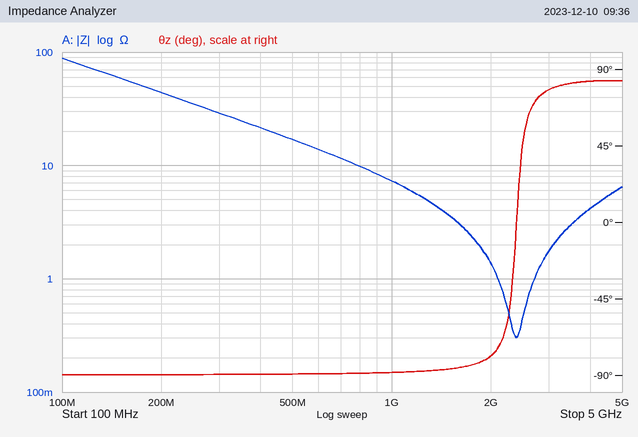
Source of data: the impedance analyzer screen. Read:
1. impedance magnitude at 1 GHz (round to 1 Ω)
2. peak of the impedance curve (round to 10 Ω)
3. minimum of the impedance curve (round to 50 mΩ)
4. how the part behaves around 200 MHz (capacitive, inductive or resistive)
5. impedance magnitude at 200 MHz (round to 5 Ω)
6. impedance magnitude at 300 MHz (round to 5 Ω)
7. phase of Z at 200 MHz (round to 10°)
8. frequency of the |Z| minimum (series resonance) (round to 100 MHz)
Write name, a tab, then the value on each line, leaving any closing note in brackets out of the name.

impedance magnitude at 1 GHz	7 Ω
peak of the impedance curve	90 Ω
minimum of the impedance curve	300 mΩ
how the part behaves around 200 MHz	capacitive
impedance magnitude at 200 MHz	45 Ω
impedance magnitude at 300 MHz	30 Ω
phase of Z at 200 MHz	-90°
frequency of the |Z| minimum (series resonance)	2.4 GHz
